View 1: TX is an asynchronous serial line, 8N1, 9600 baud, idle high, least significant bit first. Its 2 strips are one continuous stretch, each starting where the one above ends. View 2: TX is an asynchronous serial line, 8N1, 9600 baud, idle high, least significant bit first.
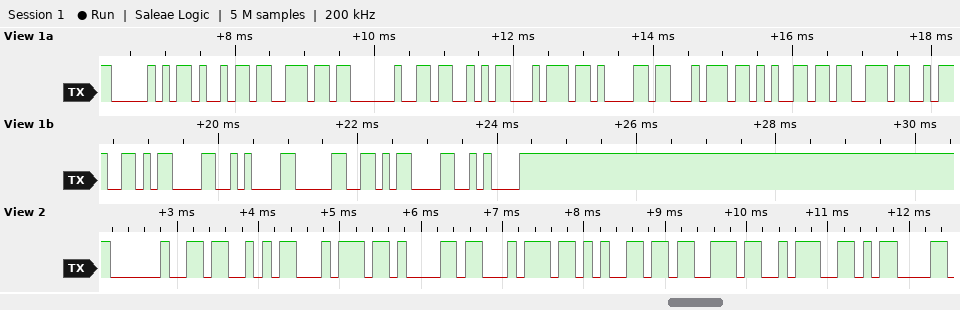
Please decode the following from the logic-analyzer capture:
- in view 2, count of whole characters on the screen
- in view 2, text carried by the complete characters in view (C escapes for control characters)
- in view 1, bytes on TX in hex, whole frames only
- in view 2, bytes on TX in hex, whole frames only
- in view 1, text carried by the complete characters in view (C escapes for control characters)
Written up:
9
" States:\r"
50 69 6E 20 53 74 61 74 65 73 3A 0D 0A 30 0D 0A
20 53 74 61 74 65 73 3A 0D
"Pin States:\r\n0\r\n"
